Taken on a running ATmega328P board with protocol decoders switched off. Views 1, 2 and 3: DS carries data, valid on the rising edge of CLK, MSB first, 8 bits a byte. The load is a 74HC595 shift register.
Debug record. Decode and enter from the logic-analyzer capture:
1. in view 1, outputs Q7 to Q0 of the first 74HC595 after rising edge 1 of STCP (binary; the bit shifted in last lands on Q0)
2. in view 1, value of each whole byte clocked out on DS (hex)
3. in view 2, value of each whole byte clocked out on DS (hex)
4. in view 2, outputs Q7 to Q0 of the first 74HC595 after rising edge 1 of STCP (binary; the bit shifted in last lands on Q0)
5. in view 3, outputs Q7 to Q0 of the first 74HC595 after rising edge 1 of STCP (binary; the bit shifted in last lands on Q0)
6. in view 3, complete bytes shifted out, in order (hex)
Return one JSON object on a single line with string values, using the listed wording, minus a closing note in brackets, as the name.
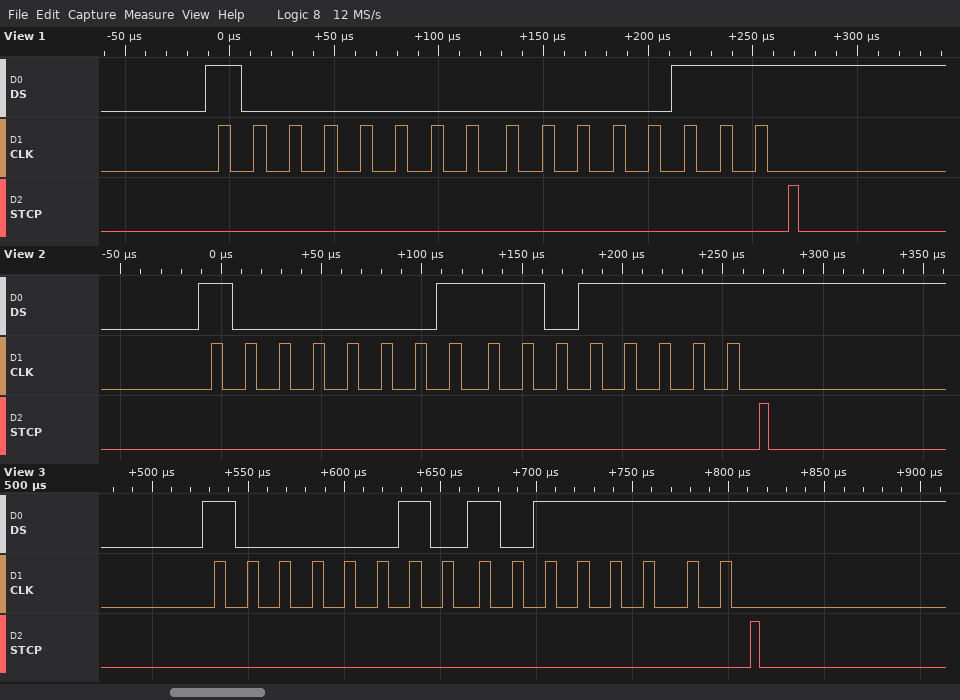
{"in view 1, outputs Q7 to Q0 of the first 74HC595 after rising edge 1 of STCP": "00000111", "in view 1, value of each whole byte clocked out on DS": "80 07", "in view 2, value of each whole byte clocked out on DS": "81 DF", "in view 2, outputs Q7 to Q0 of the first 74HC595 after rising edge 1 of STCP": "11011111", "in view 3, outputs Q7 to Q0 of the first 74HC595 after rising edge 1 of STCP": "10111111", "in view 3, complete bytes shifted out, in order": "0x82 0xBF"}
